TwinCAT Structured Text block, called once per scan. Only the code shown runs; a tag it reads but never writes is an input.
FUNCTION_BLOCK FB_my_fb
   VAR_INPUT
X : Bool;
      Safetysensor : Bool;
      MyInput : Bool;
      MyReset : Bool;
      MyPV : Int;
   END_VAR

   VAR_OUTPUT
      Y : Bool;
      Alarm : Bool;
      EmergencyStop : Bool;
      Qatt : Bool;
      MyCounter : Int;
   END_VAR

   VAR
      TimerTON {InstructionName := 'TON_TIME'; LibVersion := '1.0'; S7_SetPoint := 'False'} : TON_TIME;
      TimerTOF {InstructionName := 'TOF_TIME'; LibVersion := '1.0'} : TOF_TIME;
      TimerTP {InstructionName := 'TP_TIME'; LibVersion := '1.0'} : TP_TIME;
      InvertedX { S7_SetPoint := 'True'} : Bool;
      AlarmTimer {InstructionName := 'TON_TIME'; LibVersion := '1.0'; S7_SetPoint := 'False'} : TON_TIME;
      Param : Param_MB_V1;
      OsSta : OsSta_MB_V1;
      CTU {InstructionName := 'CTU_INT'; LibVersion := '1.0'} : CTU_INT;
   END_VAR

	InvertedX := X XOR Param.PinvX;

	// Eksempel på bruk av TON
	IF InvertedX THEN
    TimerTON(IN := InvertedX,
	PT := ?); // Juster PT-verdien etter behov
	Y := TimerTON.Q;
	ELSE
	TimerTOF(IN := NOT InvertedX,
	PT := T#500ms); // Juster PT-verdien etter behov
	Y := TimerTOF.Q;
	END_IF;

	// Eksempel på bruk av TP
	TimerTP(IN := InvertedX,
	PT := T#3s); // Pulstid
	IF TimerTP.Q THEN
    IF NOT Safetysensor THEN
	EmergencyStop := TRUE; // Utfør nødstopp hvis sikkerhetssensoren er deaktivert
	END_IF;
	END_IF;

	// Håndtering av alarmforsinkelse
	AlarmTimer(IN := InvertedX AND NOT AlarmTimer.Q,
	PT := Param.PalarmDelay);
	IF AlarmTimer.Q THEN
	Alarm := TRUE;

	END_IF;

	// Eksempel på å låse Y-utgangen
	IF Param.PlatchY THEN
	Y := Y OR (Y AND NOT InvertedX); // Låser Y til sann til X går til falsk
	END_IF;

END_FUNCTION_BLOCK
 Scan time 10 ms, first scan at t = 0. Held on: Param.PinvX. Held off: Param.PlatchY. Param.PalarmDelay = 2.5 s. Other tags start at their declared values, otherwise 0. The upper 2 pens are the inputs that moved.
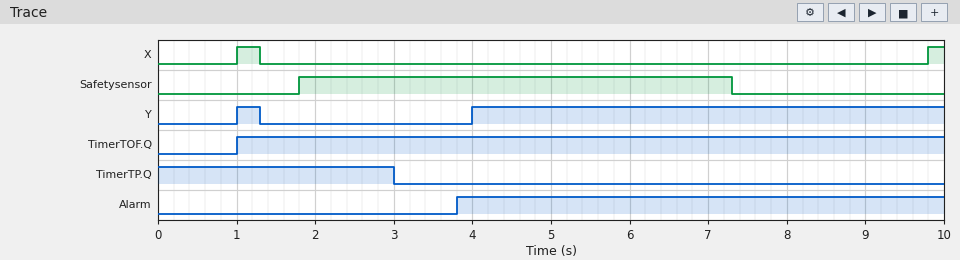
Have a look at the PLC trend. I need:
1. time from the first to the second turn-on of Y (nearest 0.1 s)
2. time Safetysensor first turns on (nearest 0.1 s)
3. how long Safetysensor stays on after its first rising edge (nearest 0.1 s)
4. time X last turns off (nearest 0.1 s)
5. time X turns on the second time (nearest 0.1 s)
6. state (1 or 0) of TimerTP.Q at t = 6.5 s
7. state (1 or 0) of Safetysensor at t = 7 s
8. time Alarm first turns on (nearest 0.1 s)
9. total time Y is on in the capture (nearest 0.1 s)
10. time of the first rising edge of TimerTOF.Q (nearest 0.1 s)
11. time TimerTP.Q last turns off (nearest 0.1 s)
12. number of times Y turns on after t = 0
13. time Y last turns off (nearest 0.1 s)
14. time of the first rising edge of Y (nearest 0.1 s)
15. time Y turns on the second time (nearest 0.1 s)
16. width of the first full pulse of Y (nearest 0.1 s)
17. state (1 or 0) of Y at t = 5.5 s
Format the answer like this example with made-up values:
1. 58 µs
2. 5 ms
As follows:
1. 3.0 s
2. 1.8 s
3. 5.5 s
4. 1.3 s
5. 9.8 s
6. 0
7. 1
8. 3.8 s
9. 6.3 s
10. 1.0 s
11. 3.0 s
12. 2
13. 1.3 s
14. 1.0 s
15. 4.0 s
16. 0.3 s
17. 1
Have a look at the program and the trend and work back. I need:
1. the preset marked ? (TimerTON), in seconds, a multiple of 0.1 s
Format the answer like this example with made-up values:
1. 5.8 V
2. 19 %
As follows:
1. 4.0 s
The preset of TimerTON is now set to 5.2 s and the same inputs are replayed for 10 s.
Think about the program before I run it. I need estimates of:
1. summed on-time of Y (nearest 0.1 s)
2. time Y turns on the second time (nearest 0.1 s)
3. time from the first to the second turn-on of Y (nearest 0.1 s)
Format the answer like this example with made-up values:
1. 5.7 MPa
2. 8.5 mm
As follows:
1. 5.1 s
2. 5.2 s
3. 4.2 s
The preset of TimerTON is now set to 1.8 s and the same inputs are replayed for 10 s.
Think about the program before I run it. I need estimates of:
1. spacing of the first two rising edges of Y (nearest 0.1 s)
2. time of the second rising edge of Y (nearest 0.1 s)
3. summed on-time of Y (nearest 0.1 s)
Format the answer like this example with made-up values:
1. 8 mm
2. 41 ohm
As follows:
1. 0.8 s
2. 1.8 s
3. 8.5 s
